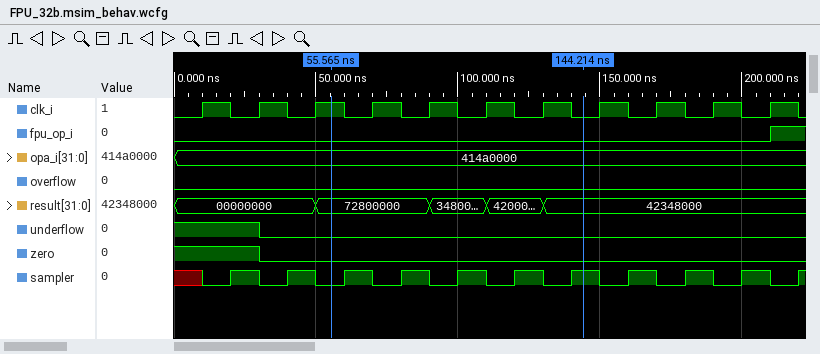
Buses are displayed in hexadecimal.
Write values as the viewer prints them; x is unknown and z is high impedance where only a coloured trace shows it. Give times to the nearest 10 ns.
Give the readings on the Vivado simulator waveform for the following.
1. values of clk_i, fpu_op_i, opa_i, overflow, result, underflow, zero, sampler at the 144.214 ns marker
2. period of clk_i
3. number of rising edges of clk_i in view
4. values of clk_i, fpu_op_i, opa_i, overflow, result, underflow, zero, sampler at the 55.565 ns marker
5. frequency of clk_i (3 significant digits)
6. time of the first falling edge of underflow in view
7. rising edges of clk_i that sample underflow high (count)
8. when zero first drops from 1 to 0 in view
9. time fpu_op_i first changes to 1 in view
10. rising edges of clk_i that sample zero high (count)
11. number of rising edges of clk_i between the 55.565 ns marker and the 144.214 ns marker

clk_i=0, fpu_op_i=0, opa_i=414a0000, overflow=0, result=42348000, underflow=0, zero=0, sampler=1
20 ns
11
clk_i=1, fpu_op_i=0, opa_i=414a0000, overflow=0, result=72800000, underflow=0, zero=0, sampler=0
50.0 MHz
30 ns
2
30 ns
210 ns
2
4
